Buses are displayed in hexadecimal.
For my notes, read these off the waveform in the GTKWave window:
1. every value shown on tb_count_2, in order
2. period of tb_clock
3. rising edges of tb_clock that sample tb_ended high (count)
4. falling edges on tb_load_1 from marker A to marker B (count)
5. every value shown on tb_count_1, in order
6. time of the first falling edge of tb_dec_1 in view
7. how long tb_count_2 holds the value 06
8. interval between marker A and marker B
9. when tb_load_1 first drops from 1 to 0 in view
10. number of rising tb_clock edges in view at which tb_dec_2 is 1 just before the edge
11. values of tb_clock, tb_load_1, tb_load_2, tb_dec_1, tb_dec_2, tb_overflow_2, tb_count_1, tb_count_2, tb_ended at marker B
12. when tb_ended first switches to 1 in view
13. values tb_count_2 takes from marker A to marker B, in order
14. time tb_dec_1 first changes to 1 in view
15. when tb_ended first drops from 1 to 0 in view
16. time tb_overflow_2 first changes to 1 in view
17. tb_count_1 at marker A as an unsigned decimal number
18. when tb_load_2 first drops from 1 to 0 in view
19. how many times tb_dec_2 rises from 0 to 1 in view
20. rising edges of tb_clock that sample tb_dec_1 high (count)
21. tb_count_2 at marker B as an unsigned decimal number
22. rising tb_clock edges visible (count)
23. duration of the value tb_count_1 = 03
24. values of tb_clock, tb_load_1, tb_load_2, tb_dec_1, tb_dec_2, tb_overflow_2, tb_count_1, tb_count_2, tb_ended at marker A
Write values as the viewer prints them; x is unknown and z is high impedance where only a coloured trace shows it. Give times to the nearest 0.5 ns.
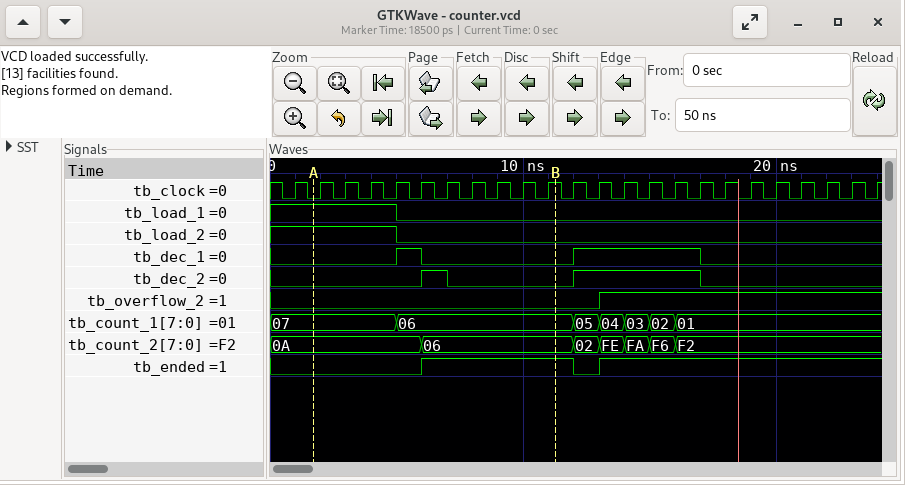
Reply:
0A, 06, 02, FE, FA, F6, F2
1 ns
17
1
07, 06, 05, 04, 03, 02, 01
6 ns
6 ns
9.5 ns
5 ns
6
tb_clock=1, tb_load_1=0, tb_load_2=0, tb_dec_1=0, tb_dec_2=0, tb_overflow_2=0, tb_count_1=06, tb_count_2=06, tb_ended=1
6 ns
0A, 06
5 ns
12 ns
13 ns
7
5 ns
2
6
6
24
1 ns
tb_clock=0, tb_load_1=1, tb_load_2=1, tb_dec_1=0, tb_dec_2=0, tb_overflow_2=0, tb_count_1=07, tb_count_2=0A, tb_ended=0
